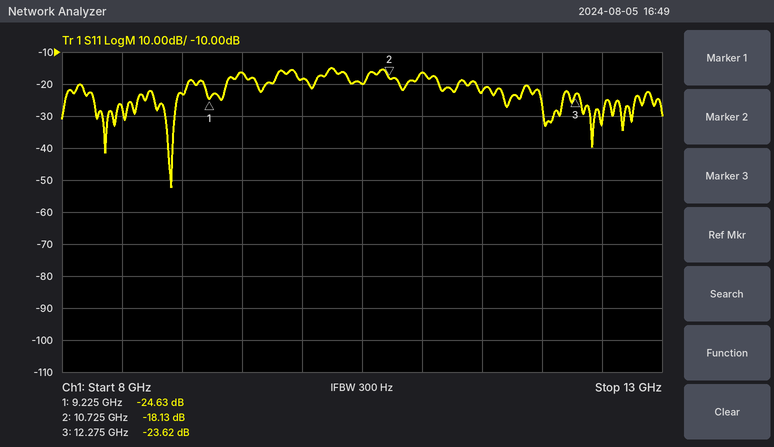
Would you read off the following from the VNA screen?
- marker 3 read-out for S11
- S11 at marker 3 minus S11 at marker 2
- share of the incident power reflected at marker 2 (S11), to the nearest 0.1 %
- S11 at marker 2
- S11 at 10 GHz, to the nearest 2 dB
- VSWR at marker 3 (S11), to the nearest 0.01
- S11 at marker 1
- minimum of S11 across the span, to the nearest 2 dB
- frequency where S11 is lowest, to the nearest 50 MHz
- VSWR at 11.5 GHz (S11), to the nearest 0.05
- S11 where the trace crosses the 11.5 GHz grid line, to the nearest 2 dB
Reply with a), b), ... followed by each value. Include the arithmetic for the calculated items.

a) -23.62 dB
b) -23.62 − (-18.13) = -5.49 dB
c) 10^(-18.13/10) ≈ 1.5 %
d) -18.13 dB
e) -18 dB
f) (1 + 0.0659)/(1 − 0.0659) ≈ 1.14
g) -24.63 dB
h) -52 dB
i) 8.90 GHz
j) |Γ| = 10^(-22/20) = 0.0794; VSWR = (1 + 0.0794)/(1 − 0.0794) ≈ 1.17, so 1.15 to the nearest 0.05
k) -22 dB
